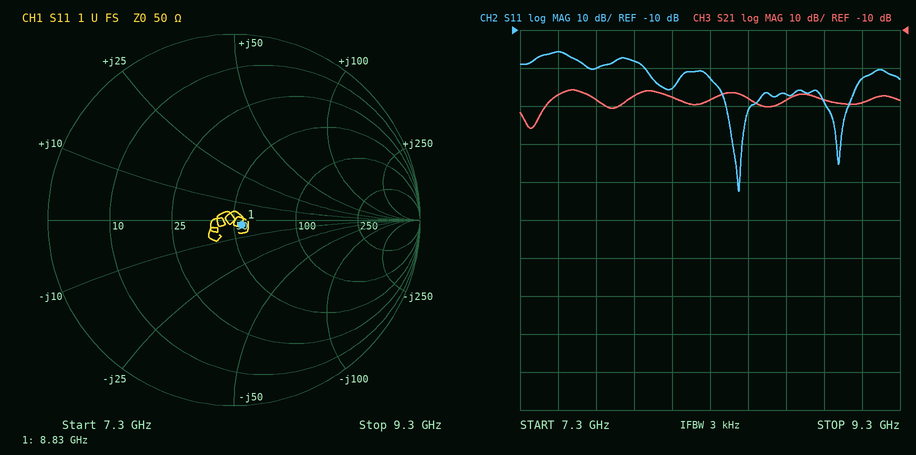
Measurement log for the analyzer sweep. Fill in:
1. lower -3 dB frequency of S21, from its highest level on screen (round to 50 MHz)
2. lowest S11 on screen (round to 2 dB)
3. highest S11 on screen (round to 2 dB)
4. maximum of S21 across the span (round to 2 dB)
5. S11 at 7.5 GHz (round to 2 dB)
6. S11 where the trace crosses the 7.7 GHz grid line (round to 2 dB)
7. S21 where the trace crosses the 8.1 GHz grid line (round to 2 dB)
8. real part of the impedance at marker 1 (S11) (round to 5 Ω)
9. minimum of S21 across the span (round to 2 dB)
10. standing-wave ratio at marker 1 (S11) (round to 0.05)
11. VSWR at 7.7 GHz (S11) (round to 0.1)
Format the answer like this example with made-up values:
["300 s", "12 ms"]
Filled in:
["7.45 GHz", "-52 dB", "-16 dB", "-26 dB", "-16 dB", "-20 dB", "-28 dB", "55 Ω", "-36 dB", "1.10", "1.2"]
